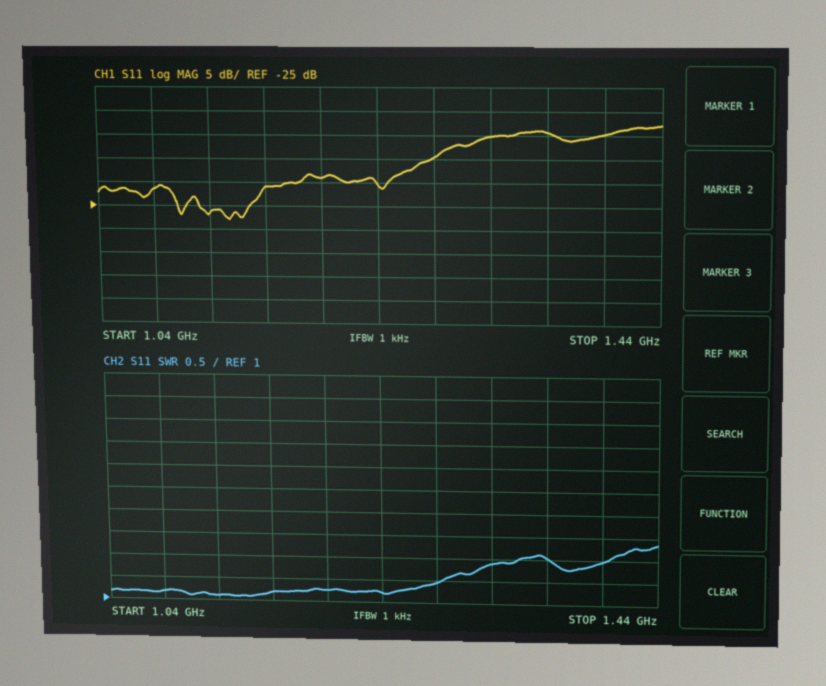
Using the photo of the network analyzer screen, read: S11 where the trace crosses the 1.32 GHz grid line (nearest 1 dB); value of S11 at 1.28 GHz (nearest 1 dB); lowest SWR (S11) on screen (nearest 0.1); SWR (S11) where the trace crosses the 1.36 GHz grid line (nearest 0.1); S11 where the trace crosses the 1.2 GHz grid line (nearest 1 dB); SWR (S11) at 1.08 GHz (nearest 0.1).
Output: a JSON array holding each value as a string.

["-10 dB", "-15 dB", "1.1", "2.0", "-19 dB", "1.2"]
